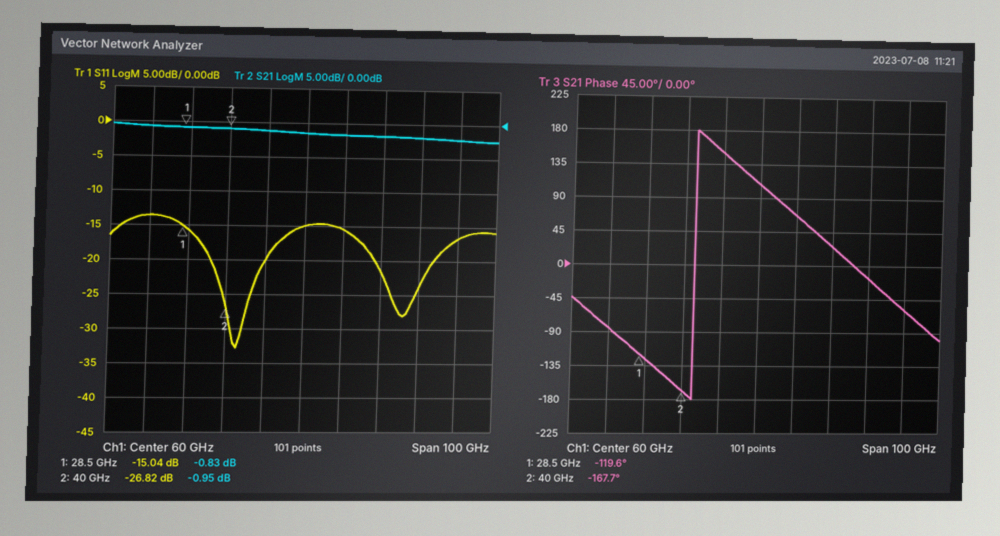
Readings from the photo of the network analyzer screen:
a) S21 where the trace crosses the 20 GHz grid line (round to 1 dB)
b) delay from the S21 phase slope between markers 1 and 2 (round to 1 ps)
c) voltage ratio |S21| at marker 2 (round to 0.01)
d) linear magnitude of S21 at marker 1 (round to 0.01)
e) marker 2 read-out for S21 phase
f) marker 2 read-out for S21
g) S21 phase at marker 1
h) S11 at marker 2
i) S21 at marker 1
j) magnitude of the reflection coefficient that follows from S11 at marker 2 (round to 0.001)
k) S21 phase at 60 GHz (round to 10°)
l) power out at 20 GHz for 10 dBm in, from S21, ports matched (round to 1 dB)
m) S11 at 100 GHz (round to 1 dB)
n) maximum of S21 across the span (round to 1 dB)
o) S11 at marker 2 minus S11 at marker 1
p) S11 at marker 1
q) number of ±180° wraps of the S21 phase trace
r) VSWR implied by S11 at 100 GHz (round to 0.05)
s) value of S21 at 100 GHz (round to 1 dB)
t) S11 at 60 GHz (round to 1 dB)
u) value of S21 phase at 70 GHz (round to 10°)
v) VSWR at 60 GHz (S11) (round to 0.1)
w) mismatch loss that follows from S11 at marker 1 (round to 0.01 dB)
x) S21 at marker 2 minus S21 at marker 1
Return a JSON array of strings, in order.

["-1 dB", "12 ps", "0.90", "0.91", "-167.7°", "-0.95 dB", "-119.6°", "-26.82 dB", "-0.83 dB", "0.046", "110°", "9 dBm", "-17 dB", "0 dB", "-11.78 dB", "-15.04 dB", "1", "1.35", "-2 dB", "-15 dB", "70°", "1.4", "0.14 dB", "-0.12 dB"]
